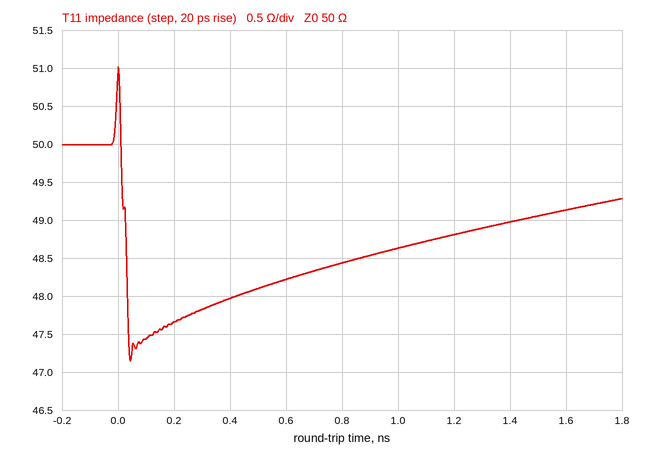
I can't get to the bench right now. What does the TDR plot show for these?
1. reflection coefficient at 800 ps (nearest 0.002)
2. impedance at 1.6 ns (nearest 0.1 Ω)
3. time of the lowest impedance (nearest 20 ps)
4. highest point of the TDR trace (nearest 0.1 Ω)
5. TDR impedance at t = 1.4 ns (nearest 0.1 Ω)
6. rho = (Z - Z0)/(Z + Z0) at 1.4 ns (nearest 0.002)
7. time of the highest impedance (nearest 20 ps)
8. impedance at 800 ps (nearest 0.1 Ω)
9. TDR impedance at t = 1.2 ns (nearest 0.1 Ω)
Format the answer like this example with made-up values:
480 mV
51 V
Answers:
-0.016
49.1 Ω
40 ps
51.0 Ω
49.0 Ω
-0.010
0 ps
48.4 Ω
48.8 Ω
